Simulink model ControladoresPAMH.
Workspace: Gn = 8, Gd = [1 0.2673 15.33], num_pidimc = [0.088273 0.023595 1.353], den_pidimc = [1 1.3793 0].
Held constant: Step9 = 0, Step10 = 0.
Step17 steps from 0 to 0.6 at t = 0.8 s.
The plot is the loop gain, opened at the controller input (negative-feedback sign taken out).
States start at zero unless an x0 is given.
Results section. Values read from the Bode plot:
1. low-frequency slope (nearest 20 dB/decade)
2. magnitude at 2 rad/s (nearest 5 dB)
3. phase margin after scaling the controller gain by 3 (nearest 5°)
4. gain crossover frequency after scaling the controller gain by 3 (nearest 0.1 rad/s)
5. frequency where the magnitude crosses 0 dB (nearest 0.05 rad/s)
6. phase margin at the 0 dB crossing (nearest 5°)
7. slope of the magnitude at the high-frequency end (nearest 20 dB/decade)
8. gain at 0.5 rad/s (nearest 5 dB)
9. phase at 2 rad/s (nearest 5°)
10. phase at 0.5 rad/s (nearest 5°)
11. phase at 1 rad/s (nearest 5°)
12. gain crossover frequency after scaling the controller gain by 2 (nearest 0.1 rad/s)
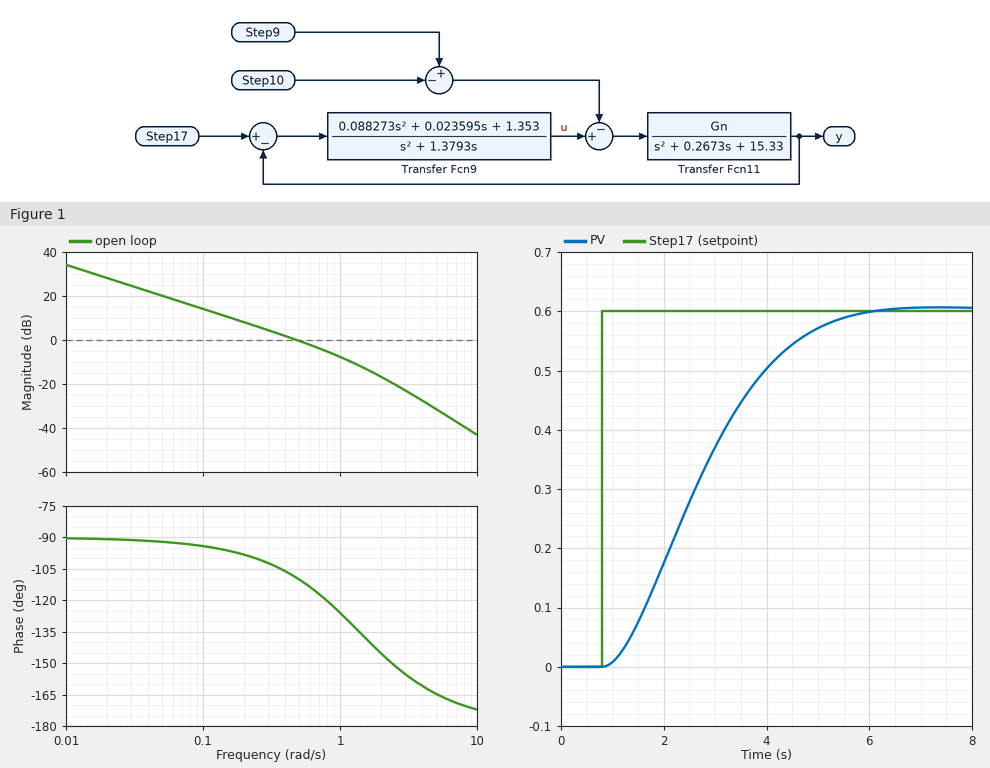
-20 dB/decade
-15 dB
50°
1.2 rad/s
0.50 rad/s
70°
-40 dB/decade
0 dB
-145°
-110°
-125°
0.9 rad/s
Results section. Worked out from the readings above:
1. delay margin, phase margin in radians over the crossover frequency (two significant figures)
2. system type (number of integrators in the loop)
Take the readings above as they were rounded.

2.4 s
1
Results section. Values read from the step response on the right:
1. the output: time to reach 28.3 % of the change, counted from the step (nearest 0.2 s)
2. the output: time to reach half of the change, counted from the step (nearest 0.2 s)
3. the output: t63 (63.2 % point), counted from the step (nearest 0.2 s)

1.2 s
1.8 s
2.2 s
